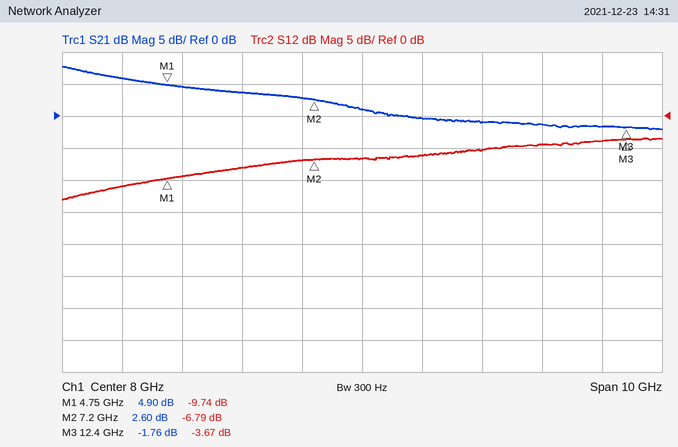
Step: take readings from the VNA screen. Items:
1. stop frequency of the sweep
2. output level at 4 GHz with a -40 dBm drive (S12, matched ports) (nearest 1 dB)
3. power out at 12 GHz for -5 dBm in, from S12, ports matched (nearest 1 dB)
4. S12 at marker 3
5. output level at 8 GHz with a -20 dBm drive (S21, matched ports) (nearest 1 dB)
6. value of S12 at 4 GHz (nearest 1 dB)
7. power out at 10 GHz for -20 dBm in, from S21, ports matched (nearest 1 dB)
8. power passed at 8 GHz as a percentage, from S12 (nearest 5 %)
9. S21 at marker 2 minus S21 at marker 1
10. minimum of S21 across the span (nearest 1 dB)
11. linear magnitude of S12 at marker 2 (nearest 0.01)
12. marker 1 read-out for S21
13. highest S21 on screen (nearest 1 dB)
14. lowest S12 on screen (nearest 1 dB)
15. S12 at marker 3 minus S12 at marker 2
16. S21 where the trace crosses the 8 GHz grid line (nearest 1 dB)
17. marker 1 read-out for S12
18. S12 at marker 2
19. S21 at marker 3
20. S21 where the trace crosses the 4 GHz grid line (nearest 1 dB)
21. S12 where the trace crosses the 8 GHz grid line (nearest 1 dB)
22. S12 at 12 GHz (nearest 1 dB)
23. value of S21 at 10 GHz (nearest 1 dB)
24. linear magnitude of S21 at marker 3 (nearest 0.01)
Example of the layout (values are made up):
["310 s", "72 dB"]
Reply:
["13 GHz", "-51 dBm", "-9 dBm", "-3.67 dB", "-19 dBm", "-11 dB", "-21 dBm", "20 %", "-2.30 dB", "-2 dB", "0.46", "4.90 dB", "8 dB", "-13 dB", "3.12 dB", "1 dB", "-9.74 dB", "-6.79 dB", "-1.76 dB", "6 dB", "-7 dB", "-4 dB", "-1 dB", "0.82"]
